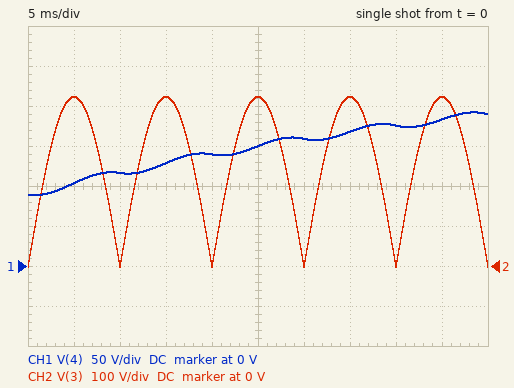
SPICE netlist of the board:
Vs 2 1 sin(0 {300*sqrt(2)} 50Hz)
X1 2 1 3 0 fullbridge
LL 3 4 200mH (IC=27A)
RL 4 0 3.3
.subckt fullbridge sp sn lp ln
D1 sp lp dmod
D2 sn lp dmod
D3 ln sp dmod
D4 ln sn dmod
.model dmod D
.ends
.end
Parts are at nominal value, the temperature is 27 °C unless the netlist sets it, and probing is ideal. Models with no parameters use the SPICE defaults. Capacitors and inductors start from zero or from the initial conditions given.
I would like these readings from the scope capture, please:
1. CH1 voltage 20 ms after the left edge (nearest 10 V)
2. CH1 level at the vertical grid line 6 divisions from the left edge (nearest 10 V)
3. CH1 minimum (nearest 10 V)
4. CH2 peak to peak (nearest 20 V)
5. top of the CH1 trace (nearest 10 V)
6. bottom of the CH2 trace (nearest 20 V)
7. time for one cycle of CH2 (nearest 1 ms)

140 V
160 V
90 V
420 V
190 V
0 V
10 ms
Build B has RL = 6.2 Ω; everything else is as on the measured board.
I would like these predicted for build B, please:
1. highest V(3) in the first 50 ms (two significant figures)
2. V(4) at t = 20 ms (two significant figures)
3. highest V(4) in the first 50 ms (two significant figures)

420 V
210 V
250 V
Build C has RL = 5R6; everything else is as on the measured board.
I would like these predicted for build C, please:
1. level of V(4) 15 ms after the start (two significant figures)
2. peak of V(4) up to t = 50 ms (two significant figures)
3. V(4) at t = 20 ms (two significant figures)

190 V
250 V
200 V
